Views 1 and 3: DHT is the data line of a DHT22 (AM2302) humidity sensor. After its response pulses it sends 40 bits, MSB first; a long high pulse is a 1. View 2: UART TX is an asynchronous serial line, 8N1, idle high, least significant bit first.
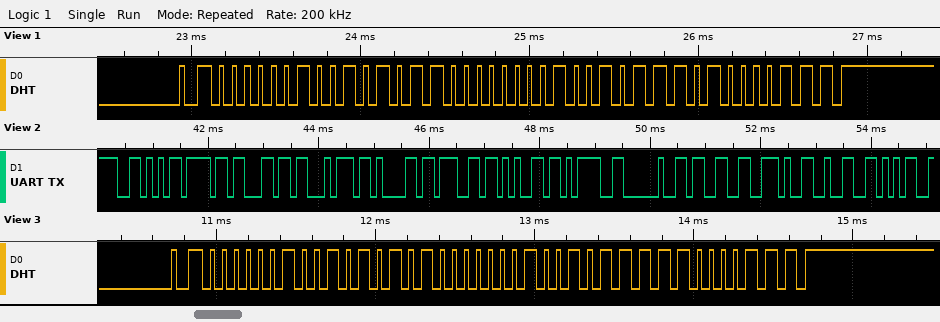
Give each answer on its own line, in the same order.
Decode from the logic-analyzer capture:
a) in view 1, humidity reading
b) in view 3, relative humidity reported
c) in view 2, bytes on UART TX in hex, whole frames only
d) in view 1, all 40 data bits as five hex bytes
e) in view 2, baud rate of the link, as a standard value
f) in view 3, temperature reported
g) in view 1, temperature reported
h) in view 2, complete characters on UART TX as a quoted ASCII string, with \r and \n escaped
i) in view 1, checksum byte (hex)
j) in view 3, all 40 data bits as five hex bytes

59.8 %
59.7 %
56 6F 6C 74 61 67 65 3D 20 33 2E 32 35
02 56 01 2E 87
9600 baud
30.3 °C
30.2 °C
"Voltage= 3.25"
0x87
02 55 01 2F 87
